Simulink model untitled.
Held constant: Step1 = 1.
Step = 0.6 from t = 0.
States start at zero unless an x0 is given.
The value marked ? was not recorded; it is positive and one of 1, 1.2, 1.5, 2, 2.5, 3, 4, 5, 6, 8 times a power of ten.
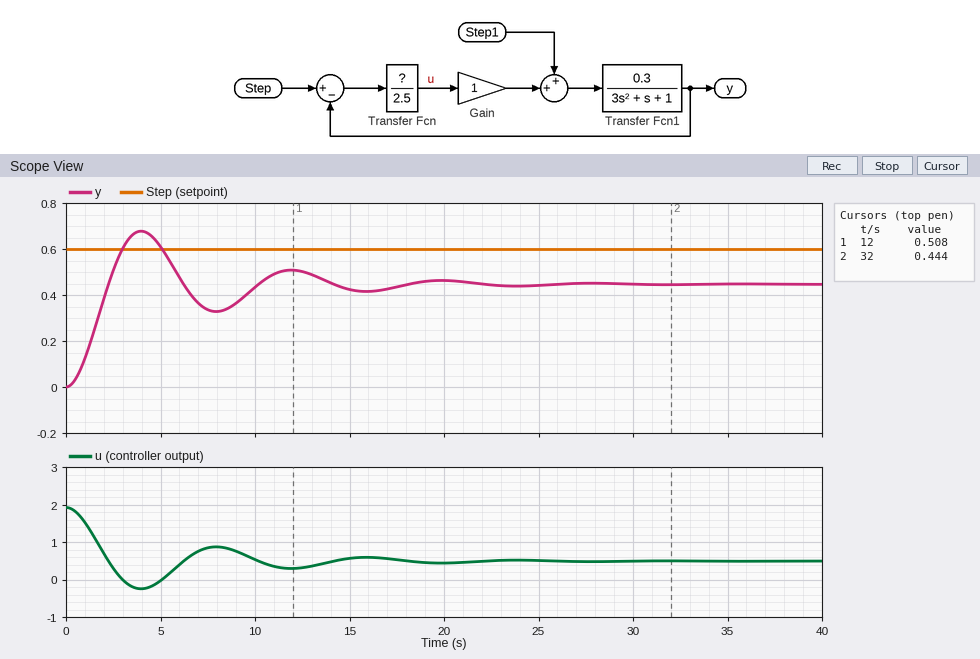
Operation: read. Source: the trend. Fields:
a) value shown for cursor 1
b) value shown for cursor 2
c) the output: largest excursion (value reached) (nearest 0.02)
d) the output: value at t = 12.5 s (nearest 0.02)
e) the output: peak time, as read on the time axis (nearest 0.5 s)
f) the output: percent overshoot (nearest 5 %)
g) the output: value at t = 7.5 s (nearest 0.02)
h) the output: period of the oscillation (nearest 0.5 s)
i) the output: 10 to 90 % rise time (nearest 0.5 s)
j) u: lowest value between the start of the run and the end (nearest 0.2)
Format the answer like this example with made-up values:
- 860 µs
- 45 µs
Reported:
- 0.508
- 0.444
- 0.68
- 0.50
- 4.0 s
- 50 %
- 0.34
- 8.0 s
- 1.5 s
- -0.2
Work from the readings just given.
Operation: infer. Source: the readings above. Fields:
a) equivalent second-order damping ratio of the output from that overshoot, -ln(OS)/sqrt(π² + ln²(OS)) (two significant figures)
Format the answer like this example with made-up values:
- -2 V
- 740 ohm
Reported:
- 0.22
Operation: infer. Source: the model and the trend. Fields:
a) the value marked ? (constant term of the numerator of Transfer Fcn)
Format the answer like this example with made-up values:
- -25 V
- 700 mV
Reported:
- 8
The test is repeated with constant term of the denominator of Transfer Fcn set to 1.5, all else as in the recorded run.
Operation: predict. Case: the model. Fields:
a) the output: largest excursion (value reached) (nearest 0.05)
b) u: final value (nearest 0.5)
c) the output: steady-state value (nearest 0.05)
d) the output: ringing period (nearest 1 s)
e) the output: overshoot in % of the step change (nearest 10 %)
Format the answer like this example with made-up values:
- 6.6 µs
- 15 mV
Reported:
- 0.75
- 0.5
- 0.50
- 7 s
- 60 %
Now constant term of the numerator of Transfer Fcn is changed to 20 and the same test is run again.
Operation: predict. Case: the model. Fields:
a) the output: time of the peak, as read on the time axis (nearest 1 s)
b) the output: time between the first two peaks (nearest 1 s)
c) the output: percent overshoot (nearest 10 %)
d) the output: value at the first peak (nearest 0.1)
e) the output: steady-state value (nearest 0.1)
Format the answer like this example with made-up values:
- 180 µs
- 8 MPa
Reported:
- 3 s
- 6 s
- 60 %
- 0.8
- 0.5
